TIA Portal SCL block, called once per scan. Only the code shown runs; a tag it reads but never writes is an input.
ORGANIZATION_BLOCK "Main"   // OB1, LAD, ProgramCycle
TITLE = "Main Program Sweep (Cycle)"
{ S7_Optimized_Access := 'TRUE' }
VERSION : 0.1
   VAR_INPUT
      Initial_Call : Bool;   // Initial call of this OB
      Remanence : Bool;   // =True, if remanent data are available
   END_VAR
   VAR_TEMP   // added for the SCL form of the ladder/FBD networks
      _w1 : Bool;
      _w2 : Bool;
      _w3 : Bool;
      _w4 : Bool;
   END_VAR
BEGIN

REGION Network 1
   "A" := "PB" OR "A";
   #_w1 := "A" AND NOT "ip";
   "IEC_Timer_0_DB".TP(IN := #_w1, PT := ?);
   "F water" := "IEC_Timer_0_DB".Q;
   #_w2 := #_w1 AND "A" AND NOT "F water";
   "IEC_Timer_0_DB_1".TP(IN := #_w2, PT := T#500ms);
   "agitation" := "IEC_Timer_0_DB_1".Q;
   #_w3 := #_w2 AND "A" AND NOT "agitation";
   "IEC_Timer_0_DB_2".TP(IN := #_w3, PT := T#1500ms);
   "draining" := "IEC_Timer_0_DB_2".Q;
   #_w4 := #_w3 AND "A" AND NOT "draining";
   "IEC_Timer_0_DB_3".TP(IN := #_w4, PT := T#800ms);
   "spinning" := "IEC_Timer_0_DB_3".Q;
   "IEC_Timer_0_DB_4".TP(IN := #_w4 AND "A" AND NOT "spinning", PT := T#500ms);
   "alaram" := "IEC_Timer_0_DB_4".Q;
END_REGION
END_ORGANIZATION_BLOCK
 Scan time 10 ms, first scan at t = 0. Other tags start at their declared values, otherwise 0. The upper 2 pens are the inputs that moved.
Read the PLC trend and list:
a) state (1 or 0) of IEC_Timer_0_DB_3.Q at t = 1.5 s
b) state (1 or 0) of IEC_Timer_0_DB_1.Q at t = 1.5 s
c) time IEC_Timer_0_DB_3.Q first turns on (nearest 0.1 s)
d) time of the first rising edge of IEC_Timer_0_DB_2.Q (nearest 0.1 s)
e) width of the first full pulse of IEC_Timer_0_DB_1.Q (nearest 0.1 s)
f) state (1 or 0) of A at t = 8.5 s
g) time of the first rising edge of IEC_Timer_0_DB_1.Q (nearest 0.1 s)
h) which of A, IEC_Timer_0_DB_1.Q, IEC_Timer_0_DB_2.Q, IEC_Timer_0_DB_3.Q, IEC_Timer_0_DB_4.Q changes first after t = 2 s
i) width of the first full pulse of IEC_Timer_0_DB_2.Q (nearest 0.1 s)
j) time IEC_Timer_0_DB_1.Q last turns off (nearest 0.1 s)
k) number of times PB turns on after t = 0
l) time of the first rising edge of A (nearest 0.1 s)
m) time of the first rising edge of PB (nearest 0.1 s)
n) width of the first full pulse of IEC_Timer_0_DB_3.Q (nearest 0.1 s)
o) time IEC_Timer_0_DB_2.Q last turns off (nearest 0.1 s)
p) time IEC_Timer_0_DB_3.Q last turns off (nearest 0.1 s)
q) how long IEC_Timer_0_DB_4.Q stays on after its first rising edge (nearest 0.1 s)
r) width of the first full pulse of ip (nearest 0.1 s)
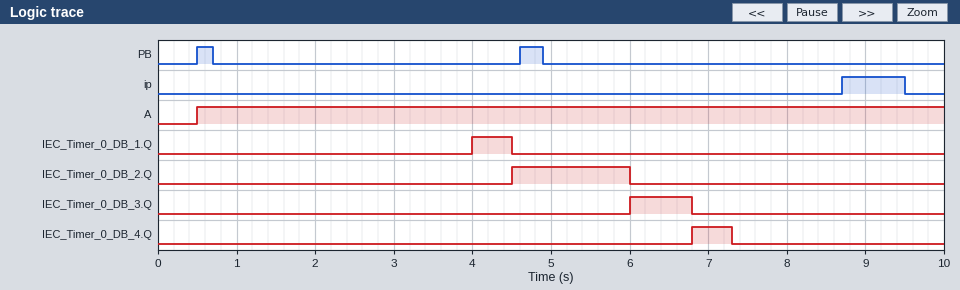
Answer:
0
0
6.0 s
4.5 s
0.5 s
1
4.0 s
IEC_Timer_0_DB_1.Q
1.5 s
4.5 s
2
0.5 s
0.5 s
0.8 s
6.0 s
6.8 s
0.5 s
0.8 s
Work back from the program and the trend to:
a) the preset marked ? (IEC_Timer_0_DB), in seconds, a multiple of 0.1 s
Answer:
3.5 s
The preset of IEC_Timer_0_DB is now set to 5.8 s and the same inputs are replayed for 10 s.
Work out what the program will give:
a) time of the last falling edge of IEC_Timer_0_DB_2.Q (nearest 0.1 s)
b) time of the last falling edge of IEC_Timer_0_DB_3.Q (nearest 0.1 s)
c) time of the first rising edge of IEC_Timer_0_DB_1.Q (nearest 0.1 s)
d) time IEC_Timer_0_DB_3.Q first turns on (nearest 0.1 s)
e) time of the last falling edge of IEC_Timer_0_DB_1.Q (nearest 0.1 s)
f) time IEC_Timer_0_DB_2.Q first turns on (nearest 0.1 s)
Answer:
8.3 s
9.1 s
6.3 s
8.3 s
6.8 s
6.8 s
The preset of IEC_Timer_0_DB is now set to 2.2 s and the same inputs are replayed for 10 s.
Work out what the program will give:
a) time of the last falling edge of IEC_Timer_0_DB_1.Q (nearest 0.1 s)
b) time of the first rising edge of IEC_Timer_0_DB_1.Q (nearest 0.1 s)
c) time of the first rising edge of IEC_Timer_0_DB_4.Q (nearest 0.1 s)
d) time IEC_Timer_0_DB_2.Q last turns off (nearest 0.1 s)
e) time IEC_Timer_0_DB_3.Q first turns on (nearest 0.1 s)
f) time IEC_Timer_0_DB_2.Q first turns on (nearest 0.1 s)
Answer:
3.2 s
2.7 s
5.5 s
4.7 s
4.7 s
3.2 s
